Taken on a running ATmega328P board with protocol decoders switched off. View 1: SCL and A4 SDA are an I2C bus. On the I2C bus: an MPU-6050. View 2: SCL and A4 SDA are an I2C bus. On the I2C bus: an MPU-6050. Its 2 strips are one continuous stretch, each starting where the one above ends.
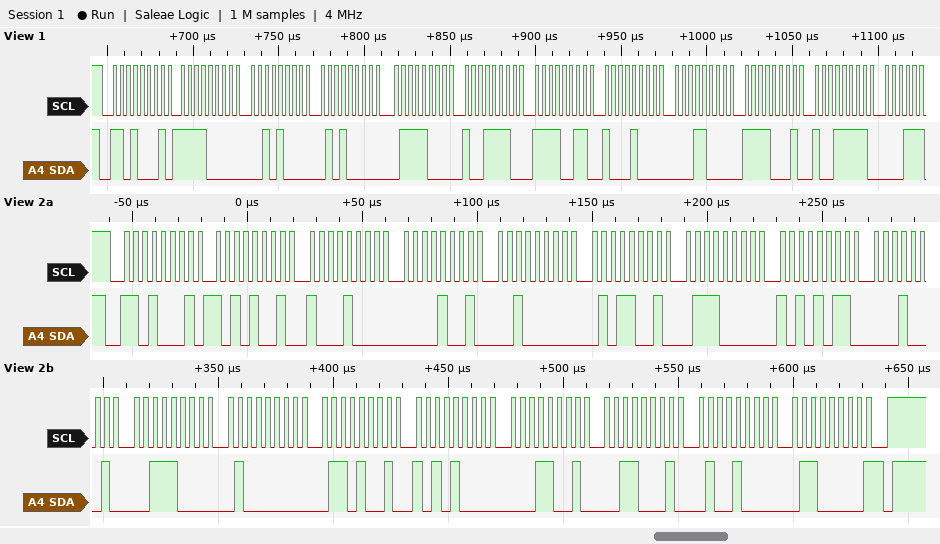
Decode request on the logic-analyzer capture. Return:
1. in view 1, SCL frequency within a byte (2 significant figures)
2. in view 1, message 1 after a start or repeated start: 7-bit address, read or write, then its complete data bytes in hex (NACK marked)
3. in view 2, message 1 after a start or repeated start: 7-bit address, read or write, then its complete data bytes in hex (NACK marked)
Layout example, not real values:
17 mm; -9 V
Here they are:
250 kHz; 0x68 read: F0 28 50 78 9E F3 88 18 F1 9F; 0x68 read: A9 88 09 20 59 70 AB 11 38 40 69 A8 19 31 48 60 NACK
